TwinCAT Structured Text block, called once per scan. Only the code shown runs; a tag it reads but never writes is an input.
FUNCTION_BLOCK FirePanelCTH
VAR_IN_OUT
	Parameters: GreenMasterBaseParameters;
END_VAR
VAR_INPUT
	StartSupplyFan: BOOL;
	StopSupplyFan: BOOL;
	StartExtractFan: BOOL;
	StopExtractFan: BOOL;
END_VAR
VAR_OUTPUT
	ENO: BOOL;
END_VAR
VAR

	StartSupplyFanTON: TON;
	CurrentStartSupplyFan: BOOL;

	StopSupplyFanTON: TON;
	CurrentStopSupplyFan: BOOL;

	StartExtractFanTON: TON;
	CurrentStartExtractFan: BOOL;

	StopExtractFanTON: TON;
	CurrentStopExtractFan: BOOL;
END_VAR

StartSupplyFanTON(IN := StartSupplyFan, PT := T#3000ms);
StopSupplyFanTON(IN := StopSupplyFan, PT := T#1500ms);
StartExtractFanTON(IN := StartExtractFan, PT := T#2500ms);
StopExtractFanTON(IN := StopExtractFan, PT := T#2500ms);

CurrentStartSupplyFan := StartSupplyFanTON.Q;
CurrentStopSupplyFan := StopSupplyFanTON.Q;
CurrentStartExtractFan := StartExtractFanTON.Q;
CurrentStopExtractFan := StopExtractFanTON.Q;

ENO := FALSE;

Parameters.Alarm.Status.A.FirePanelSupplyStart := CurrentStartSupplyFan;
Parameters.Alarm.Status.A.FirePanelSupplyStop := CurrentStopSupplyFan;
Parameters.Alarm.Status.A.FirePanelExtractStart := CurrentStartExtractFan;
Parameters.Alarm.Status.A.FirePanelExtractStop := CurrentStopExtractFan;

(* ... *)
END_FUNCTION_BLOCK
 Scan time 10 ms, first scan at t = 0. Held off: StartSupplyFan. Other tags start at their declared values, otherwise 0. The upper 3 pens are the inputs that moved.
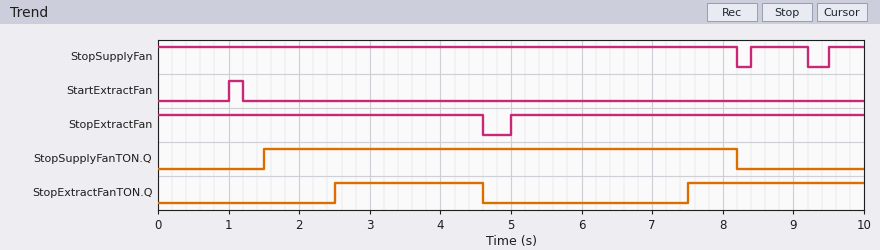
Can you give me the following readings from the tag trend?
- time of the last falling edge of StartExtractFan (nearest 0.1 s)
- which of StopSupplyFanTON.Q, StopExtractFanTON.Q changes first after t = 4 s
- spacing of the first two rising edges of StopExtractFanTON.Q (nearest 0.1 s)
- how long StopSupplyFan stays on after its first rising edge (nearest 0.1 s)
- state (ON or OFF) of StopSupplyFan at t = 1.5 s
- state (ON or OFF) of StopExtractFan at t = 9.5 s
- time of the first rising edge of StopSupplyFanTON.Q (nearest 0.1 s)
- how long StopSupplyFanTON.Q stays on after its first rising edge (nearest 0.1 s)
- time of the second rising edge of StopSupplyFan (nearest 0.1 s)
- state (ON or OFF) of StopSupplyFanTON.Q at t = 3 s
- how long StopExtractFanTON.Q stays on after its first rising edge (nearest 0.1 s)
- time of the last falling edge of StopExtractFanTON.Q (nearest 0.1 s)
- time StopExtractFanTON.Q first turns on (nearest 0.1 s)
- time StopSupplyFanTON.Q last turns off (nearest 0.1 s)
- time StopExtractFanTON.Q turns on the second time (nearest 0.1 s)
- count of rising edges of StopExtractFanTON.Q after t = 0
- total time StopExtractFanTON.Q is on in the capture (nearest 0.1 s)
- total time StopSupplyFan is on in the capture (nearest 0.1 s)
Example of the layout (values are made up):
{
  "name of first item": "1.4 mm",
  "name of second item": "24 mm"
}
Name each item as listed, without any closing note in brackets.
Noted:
{
  "time of the last falling edge of StartExtractFan": "1.2 s",
  "which of StopSupplyFanTON.Q, StopExtractFanTON.Q changes first after t = 4 s": "StopExtractFanTON.Q",
  "spacing of the first two rising edges of StopExtractFanTON.Q": "5.0 s",
  "how long StopSupplyFan stays on after its first rising edge": "0.8 s",
  "state (ON or OFF) of StopSupplyFan at t = 1.5 s": "ON",
  "state (ON or OFF) of StopExtractFan at t = 9.5 s": "ON",
  "time of the first rising edge of StopSupplyFanTON.Q": "1.5 s",
  "how long StopSupplyFanTON.Q stays on after its first rising edge": "6.7 s",
  "time of the second rising edge of StopSupplyFan": "9.5 s",
  "state (ON or OFF) of StopSupplyFanTON.Q at t = 3 s": "ON",
  "how long StopExtractFanTON.Q stays on after its first rising edge": "2.1 s",
  "time of the last falling edge of StopExtractFanTON.Q": "4.6 s",
  "time StopExtractFanTON.Q first turns on": "2.5 s",
  "time StopSupplyFanTON.Q last turns off": "8.2 s",
  "time StopExtractFanTON.Q turns on the second time": "7.5 s",
  "count of rising edges of StopExtractFanTON.Q after t = 0": "2",
  "total time StopExtractFanTON.Q is on in the capture": "4.6 s",
  "total time StopSupplyFan is on in the capture": "9.5 s"
}
